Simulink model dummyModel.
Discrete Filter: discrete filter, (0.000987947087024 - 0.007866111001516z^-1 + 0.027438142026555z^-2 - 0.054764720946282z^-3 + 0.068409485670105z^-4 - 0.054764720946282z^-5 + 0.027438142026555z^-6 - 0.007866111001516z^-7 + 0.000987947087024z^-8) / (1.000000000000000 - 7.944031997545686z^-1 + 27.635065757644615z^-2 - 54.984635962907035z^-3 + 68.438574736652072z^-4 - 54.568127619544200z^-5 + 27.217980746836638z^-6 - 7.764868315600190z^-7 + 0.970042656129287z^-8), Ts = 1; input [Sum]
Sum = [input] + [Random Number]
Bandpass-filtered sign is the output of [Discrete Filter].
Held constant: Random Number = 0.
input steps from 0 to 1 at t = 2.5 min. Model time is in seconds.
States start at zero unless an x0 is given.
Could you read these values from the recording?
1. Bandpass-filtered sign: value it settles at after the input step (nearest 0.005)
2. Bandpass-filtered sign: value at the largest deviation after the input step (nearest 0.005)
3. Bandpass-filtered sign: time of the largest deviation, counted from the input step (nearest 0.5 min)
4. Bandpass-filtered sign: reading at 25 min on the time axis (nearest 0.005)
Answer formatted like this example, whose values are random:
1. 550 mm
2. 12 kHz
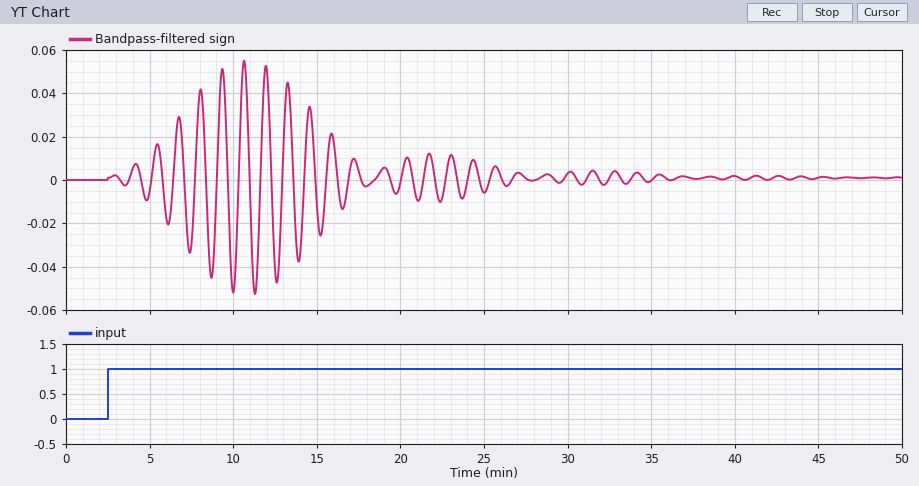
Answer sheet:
1. 0.000
2. 0.055
3. 8.0 min
4. -0.005
